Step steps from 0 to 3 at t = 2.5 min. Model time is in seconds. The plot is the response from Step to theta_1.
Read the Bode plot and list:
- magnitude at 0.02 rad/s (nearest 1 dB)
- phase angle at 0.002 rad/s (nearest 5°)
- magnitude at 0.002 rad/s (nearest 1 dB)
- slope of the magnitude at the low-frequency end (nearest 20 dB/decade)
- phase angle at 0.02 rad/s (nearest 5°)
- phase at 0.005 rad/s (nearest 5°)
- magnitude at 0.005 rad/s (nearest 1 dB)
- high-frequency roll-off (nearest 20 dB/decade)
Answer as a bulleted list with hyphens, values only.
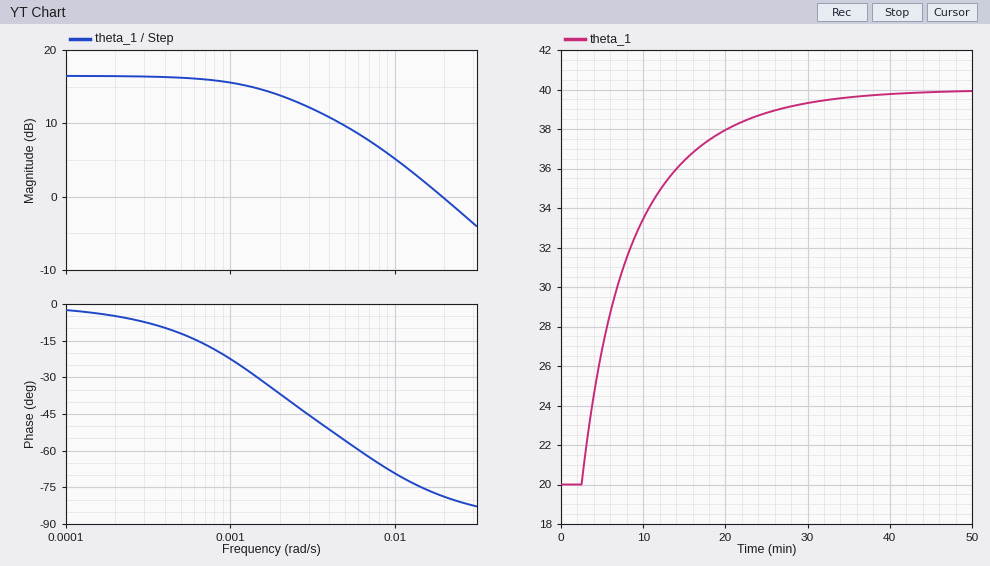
- 0 dB
- -35°
- 14 dB
- 0 dB/decade
- -80°
- -55°
- 10 dB
- -20 dB/decade
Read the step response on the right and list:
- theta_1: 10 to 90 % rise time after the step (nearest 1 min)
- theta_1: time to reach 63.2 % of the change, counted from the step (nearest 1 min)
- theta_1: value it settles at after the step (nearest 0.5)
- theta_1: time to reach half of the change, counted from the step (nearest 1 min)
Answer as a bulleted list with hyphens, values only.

- 17 min
- 7 min
- 40.0
- 4 min
